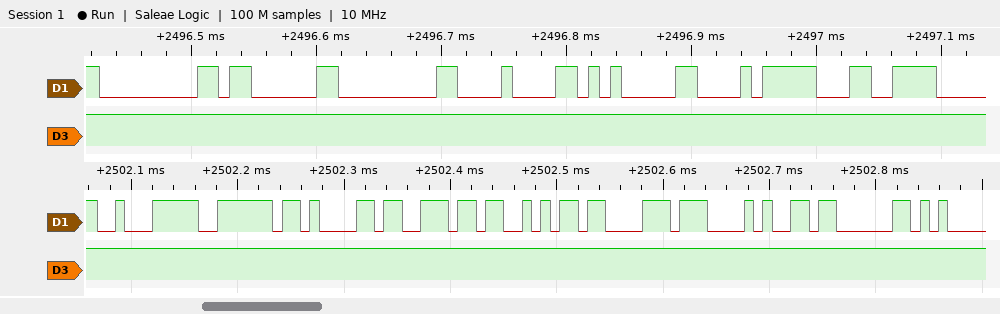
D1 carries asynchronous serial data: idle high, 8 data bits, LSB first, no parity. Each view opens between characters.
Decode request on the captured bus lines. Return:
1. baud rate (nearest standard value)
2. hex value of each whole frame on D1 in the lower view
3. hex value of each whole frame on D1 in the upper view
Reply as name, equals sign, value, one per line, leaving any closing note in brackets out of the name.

baud rate = 115200 baud
hex value of each whole frame on D1 in the lower view = E2, 7E, 61, 6E, 6A, B8, 28, 03
hex value of each whole frame on D1 in the upper view = 00, 03, 00, 08, 05, E8, CC
